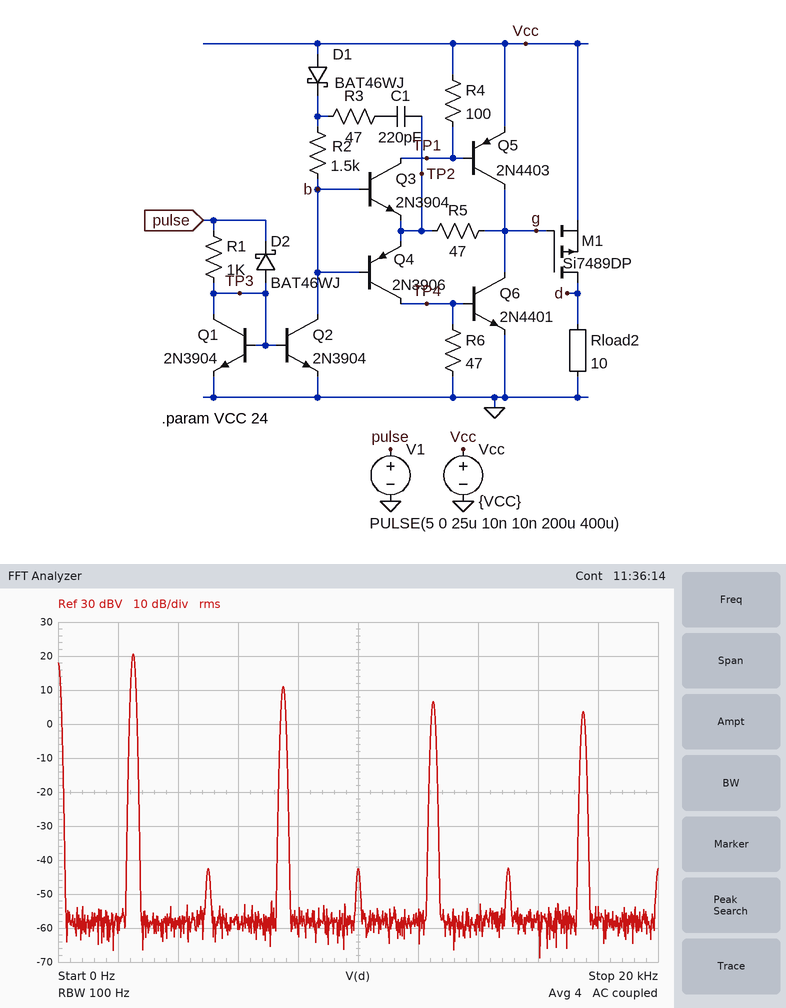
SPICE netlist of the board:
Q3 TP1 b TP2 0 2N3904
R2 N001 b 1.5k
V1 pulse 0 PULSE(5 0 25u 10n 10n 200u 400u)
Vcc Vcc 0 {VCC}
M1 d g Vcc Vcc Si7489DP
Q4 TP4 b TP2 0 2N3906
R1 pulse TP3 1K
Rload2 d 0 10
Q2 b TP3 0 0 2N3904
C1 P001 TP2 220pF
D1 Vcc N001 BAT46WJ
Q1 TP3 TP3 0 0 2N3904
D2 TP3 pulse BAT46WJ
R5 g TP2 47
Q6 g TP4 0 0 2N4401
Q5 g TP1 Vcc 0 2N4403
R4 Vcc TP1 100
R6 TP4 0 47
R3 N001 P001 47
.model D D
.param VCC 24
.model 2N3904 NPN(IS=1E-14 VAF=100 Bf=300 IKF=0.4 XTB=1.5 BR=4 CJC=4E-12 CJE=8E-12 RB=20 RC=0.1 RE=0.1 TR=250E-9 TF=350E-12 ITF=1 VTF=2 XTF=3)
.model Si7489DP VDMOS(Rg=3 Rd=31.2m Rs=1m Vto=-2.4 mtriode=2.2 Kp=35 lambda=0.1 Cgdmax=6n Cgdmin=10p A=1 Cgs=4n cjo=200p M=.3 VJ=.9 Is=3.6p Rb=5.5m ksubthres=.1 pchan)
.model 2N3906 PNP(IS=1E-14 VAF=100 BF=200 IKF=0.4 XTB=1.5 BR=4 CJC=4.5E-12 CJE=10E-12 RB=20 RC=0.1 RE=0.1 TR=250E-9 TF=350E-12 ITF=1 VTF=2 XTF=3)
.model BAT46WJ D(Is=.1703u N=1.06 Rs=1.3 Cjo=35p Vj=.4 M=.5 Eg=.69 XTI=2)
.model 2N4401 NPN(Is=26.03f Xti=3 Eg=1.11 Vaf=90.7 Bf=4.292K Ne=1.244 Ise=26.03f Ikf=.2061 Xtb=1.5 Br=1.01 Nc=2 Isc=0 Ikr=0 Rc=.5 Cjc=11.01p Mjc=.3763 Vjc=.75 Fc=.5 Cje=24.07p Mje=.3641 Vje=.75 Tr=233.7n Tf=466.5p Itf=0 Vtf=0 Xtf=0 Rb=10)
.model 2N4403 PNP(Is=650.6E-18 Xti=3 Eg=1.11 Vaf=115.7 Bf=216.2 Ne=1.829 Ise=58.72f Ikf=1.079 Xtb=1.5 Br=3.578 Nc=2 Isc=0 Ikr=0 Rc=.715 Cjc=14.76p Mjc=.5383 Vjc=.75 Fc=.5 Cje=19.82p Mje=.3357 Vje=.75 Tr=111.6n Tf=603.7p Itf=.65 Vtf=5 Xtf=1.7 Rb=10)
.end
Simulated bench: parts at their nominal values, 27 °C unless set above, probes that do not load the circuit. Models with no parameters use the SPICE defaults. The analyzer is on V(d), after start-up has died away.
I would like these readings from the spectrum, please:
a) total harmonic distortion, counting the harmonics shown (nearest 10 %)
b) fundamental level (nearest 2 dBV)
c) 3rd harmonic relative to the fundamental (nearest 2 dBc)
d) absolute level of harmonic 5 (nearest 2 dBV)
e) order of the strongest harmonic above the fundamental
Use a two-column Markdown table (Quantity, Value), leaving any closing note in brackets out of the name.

| Quantity | Value |
|---|---|
| total harmonic distortion, counting the harmonics shown | 40 % |
| fundamental level | 20 dBV |
| 3rd harmonic relative to the fundamental | -10 dBc |
| absolute level of harmonic 5 | 6 dBV |
| order of the strongest harmonic above the fundamental | 3 |
